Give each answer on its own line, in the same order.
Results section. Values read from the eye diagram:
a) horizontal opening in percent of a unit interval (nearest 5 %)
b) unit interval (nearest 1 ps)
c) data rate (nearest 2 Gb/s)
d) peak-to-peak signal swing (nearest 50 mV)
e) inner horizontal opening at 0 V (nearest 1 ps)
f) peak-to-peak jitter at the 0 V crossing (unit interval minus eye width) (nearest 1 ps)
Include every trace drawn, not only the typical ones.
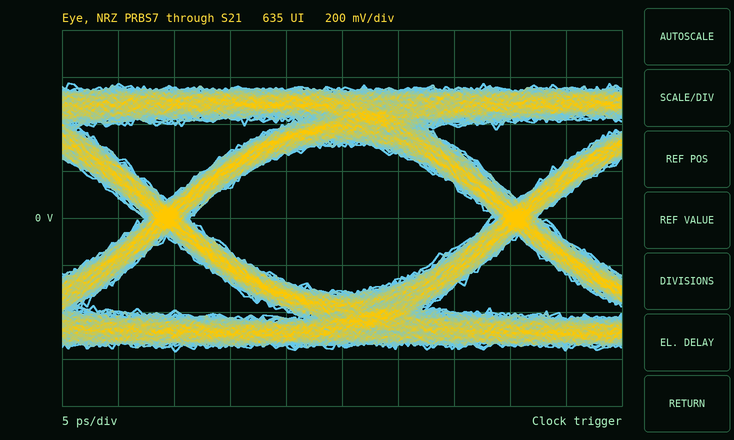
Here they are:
85 %
31 ps
32 Gb/s
1.15 V
27 ps
4 ps
